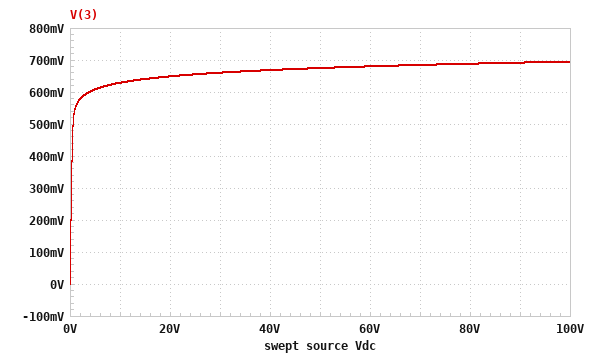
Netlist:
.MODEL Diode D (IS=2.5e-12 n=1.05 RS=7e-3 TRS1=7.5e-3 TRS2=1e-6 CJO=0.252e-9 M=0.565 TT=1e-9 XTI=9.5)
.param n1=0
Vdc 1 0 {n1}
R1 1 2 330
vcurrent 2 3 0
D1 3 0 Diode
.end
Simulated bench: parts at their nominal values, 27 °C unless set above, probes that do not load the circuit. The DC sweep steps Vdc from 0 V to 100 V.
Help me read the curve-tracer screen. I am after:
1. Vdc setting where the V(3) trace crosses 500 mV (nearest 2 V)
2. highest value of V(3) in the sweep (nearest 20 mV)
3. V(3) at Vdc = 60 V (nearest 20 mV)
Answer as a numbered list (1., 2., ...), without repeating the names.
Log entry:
1. 0 V
2. 700 mV
3. 680 mV
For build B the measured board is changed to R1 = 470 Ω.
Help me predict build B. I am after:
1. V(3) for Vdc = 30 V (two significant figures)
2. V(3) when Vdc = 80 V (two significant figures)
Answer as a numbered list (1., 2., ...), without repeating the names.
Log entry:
1. 650 mV
2. 680 mV
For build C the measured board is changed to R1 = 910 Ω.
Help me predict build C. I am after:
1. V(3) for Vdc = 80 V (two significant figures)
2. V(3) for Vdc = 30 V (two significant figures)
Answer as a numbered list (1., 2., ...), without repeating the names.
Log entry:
1. 660 mV
2. 630 mV
